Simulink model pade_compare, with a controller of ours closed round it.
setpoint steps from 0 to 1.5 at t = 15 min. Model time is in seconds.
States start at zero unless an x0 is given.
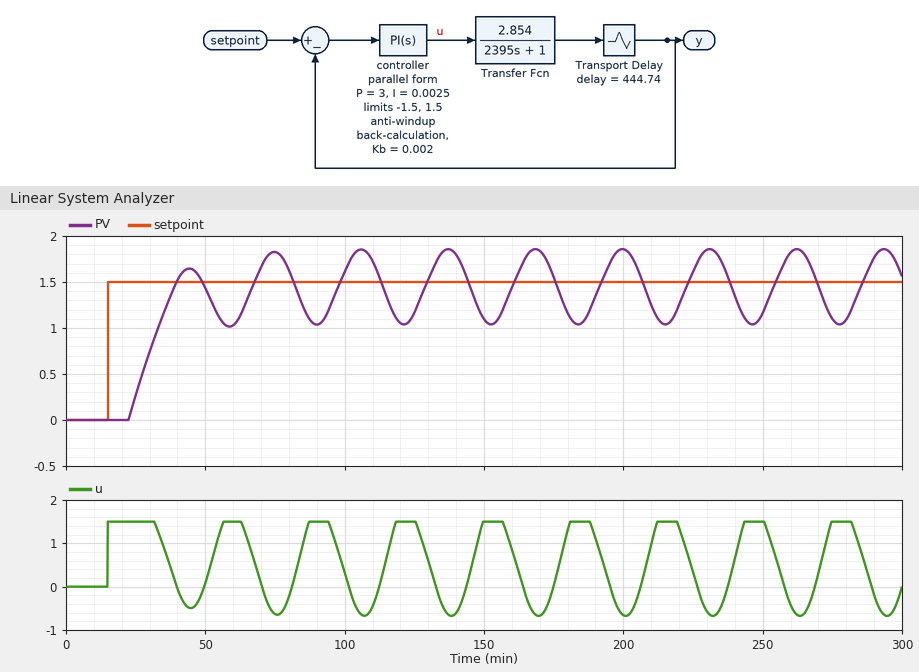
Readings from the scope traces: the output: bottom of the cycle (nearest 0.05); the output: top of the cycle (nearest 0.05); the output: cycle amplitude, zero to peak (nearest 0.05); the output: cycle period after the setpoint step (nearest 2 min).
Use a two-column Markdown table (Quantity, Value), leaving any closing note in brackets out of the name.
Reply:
| Quantity | Value |
|---|---|
| the output: bottom of the cycle | 1.05 |
| the output: top of the cycle | 1.85 |
| the output: cycle amplitude, zero to peak | 0.40 |
| the output: cycle period after the setpoint step | 32 min |
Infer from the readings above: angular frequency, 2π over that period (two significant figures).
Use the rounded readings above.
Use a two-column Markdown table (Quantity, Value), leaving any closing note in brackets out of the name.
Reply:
| Quantity | Value |
|---|---|
| angular frequency, 2π over that period | 0.20 rad/min |
